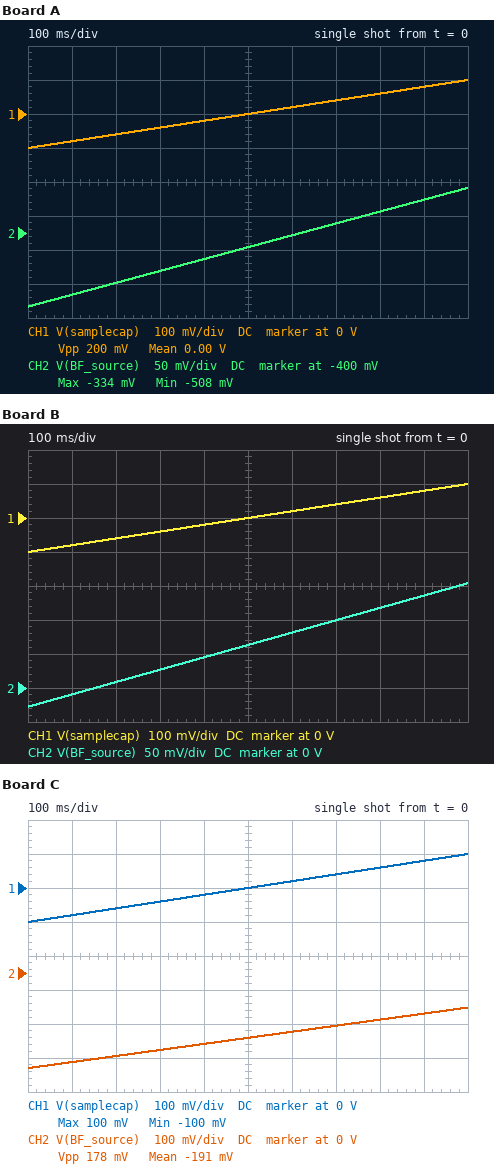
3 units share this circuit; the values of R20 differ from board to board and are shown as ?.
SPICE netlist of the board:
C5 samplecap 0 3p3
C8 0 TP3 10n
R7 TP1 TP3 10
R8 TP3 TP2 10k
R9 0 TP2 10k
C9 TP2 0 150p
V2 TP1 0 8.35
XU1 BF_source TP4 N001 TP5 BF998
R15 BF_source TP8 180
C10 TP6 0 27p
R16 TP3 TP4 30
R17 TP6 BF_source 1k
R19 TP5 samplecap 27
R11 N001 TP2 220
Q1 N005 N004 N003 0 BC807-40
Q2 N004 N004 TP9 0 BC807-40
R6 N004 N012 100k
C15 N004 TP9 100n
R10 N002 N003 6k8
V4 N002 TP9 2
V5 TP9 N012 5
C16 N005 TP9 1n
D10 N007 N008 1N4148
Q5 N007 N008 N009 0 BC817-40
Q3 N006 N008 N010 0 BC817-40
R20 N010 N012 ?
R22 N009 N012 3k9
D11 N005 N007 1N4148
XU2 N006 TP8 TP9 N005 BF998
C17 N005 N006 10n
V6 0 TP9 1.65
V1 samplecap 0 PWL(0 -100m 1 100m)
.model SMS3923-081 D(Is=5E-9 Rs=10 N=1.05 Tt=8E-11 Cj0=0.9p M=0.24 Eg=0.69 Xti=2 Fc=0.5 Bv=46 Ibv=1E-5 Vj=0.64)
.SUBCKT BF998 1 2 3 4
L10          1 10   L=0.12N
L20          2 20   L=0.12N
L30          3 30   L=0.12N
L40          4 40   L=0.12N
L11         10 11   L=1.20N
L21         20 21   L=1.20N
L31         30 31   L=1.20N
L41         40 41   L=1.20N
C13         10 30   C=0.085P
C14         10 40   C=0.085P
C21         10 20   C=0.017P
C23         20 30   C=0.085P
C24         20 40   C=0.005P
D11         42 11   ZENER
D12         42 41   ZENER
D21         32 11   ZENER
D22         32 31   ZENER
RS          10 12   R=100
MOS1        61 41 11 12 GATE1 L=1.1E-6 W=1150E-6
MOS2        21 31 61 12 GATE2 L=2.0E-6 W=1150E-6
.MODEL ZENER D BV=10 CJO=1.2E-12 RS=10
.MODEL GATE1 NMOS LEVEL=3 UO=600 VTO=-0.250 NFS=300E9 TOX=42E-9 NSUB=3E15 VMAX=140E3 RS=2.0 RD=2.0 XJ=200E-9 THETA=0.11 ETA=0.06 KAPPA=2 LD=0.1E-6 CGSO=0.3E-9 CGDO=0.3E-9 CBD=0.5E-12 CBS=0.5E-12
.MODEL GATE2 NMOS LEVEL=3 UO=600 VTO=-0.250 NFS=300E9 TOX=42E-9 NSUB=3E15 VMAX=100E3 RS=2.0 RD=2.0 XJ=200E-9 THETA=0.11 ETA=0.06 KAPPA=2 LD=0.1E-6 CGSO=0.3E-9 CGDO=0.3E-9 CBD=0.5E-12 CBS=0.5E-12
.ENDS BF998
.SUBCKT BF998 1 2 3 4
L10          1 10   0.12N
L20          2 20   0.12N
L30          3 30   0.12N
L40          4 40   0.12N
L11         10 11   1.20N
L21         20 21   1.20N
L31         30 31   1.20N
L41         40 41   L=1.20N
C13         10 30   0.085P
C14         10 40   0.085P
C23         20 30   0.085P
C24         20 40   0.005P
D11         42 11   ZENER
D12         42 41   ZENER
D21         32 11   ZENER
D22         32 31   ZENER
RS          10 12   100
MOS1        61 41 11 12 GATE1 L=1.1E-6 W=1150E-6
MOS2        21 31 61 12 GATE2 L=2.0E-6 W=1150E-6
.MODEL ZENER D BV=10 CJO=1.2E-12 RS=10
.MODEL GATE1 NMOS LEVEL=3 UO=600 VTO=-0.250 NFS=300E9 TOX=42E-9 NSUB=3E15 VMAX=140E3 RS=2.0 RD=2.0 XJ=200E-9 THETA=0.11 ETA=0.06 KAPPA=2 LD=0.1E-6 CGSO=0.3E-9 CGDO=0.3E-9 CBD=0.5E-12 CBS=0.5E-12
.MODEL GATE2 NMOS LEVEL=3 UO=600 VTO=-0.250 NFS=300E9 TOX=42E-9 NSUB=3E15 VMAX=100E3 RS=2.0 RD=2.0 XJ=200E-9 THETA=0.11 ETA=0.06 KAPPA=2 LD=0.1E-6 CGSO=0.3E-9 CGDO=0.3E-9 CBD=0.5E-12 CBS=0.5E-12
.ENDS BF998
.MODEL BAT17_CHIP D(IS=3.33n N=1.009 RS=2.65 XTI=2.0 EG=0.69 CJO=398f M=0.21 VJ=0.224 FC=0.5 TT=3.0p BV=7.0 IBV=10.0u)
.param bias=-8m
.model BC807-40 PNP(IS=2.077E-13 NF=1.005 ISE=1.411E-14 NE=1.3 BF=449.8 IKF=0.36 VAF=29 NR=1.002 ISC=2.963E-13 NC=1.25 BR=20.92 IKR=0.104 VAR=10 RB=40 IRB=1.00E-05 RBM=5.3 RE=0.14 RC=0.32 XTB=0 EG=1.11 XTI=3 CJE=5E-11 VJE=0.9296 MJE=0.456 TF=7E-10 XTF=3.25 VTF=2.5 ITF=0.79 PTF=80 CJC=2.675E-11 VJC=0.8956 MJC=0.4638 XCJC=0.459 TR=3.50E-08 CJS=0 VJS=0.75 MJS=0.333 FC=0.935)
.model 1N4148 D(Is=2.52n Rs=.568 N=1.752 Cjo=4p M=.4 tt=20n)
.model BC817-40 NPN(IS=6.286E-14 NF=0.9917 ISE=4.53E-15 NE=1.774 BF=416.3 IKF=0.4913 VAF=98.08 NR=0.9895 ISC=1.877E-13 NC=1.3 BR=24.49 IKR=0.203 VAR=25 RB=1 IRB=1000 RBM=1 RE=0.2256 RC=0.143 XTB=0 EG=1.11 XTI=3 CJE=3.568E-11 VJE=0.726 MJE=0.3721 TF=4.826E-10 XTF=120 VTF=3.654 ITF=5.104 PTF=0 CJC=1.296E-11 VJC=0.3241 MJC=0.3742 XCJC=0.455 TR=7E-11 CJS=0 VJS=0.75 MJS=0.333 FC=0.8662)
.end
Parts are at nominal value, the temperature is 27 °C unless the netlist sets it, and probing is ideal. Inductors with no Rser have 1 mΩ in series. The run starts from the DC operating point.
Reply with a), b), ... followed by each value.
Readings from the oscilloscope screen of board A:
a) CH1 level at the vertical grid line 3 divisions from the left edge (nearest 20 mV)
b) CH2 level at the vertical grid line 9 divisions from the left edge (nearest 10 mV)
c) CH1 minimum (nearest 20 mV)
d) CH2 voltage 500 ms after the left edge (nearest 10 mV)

a) -40 mV
b) -350 mV
c) -100 mV
d) -420 mV
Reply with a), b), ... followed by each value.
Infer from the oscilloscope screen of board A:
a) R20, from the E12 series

a) 33 Ω
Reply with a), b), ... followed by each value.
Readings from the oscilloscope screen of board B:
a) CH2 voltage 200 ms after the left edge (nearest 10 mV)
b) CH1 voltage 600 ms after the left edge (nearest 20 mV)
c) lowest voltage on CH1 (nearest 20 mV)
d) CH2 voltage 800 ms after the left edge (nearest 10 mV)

a) 10 mV
b) 20 mV
c) -100 mV
d) 120 mV
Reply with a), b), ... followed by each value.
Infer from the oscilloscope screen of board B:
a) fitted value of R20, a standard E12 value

a) 120 Ω
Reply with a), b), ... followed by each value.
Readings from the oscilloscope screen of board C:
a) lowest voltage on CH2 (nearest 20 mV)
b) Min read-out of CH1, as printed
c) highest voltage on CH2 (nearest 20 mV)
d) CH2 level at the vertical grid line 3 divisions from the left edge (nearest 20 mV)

a) -280 mV
b) -100 mV
c) -100 mV
d) -220 mV
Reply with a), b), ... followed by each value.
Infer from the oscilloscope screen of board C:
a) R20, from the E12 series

a) 56 Ω
